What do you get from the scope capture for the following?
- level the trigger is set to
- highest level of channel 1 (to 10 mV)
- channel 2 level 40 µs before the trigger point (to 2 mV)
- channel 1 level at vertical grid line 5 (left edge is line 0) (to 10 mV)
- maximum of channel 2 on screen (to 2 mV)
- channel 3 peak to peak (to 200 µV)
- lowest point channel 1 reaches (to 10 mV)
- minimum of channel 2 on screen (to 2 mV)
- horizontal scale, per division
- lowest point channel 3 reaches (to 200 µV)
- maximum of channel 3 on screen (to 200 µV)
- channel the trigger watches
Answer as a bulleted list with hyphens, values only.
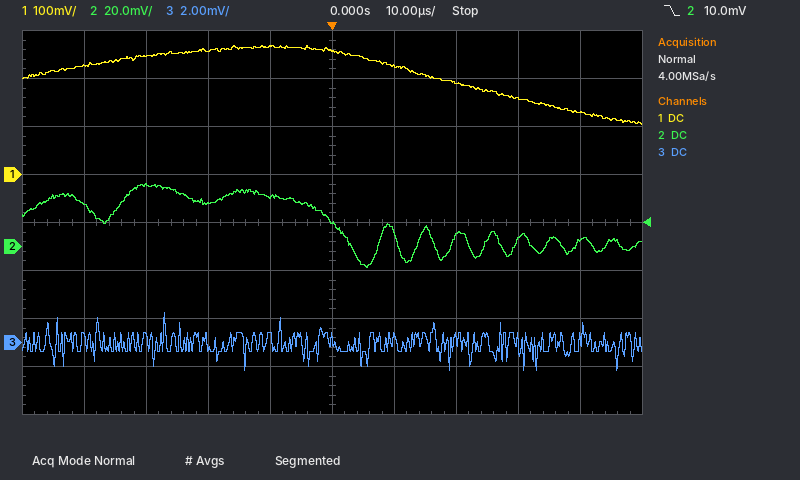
- 10.0 mV
- 270 mV
- 18 mV
- 260 mV
- 26 mV
- 2.4 mV
- 100 mV
- -8 mV
- 10 µs
- -1.2 mV
- 1.2 mV
- channel 2
